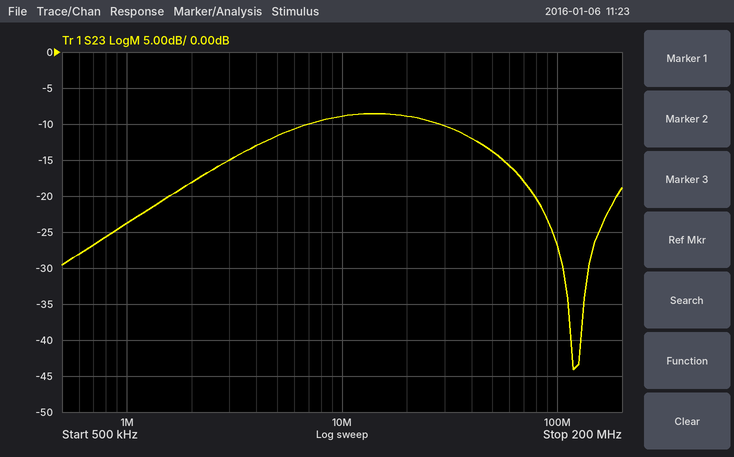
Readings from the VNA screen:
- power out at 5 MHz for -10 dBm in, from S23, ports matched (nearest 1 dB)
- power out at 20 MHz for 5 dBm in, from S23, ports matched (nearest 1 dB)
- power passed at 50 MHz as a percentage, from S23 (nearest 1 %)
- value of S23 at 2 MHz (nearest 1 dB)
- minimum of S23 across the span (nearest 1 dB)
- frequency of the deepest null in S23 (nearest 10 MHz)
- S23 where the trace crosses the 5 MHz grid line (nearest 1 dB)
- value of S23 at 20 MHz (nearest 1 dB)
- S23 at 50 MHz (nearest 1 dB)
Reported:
-22 dBm
-4 dBm
4 %
-18 dB
-44 dB
120 MHz
-12 dB
-9 dB
-14 dB
